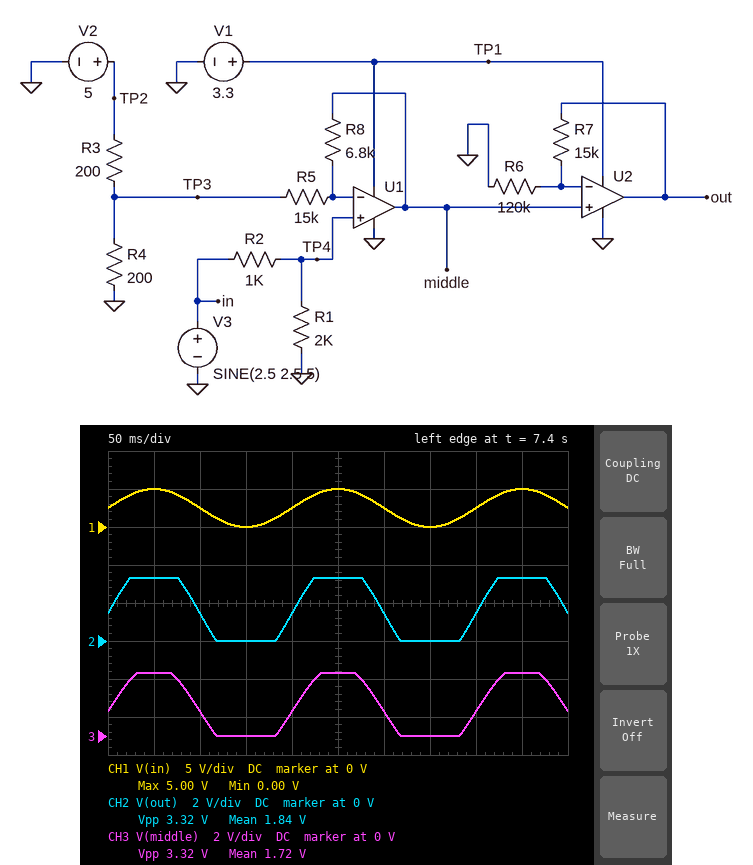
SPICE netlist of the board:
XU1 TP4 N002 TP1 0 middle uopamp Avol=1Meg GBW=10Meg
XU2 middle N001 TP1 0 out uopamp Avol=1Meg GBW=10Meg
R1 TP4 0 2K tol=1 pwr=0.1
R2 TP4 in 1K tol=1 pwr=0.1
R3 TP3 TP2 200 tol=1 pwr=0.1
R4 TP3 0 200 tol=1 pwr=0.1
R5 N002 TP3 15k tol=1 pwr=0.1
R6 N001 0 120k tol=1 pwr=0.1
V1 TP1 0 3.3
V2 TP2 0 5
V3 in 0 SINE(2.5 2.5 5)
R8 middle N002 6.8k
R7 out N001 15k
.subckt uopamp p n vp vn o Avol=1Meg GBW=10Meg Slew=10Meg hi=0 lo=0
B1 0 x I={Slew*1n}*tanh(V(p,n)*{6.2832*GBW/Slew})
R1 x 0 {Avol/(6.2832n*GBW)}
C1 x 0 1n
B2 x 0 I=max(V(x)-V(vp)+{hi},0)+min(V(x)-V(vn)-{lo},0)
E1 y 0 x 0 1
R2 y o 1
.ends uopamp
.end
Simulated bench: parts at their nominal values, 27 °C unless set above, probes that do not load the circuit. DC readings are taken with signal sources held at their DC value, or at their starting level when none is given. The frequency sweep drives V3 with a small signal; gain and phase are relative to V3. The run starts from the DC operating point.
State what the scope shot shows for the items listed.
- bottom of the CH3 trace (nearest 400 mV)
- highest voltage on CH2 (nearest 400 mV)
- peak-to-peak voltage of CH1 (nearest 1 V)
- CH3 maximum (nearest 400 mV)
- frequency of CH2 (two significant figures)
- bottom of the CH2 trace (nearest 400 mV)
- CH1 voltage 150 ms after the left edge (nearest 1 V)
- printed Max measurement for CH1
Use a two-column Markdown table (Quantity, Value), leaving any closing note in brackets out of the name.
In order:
| Quantity | Value |
|---|---|
| bottom of the CH3 trace | 0 V |
| highest voltage on CH2 | 3.2 V |
| peak-to-peak voltage of CH1 | 5 V |
| CH3 maximum | 3.2 V |
| frequency of CH2 | 5.0 Hz |
| bottom of the CH2 trace | 0 V |
| CH1 voltage 150 ms after the left edge | 0 V |
| printed Max measurement for CH1 | 5.00 V |
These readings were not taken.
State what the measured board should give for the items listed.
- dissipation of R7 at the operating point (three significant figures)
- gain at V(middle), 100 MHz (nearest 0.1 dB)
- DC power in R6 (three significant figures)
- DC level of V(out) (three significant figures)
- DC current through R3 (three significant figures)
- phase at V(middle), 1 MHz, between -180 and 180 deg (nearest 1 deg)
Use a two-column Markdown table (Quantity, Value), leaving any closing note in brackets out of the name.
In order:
| Quantity | Value |
|---|---|
| dissipation of R7 at the operating point | 1.74 µW |
| gain at V(middle), 100 MHz | -23.5 dB |
| DC power in R6 | 13.9 µW |
| DC level of V(out) | 1.45 V |
| DC current through R3 | 12.5 mA |
| phase at V(middle), 1 MHz, between -180 and 180 deg | -8 deg |
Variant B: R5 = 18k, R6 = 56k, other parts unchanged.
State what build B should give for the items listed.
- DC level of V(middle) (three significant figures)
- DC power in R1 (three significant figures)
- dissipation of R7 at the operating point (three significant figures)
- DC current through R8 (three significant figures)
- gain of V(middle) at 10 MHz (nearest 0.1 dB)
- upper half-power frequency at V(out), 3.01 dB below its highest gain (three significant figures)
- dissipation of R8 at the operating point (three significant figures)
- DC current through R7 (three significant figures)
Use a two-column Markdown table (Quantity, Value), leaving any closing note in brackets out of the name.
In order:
| Quantity | Value |
|---|---|
| DC level of V(middle) | 1.35 V |
| DC power in R1 | 1.39 mW |
| dissipation of R7 at the operating point | 8.76 µW |
| DC current through R8 | 46.0 µA |
| gain of V(middle) at 10 MHz | -5.4 dB |
| upper half-power frequency at V(out), 3.01 dB below its highest gain | 4.87 MHz |
| dissipation of R8 at the operating point | 14.4 µW |
| DC current through R7 | 24.2 µA |
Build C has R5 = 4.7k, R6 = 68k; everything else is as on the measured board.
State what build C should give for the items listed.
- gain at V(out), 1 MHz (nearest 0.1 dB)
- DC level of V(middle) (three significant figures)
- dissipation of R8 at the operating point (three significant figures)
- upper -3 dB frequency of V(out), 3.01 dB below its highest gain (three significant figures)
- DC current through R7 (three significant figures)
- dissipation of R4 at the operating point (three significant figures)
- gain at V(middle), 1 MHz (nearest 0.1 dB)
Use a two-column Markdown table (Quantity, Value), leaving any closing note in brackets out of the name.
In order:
| Quantity | Value |
|---|---|
| gain at V(out), 1 MHz | 5.6 dB |
| DC level of V(middle) | 486 mV |
| dissipation of R8 at the operating point | 205 µW |
| upper -3 dB frequency of V(out), 3.01 dB below its highest gain | 3.46 MHz |
| DC current through R7 | 7.15 µA |
| dissipation of R4 at the operating point | 30.8 mW |
| gain at V(middle), 1 MHz | 3.9 dB |
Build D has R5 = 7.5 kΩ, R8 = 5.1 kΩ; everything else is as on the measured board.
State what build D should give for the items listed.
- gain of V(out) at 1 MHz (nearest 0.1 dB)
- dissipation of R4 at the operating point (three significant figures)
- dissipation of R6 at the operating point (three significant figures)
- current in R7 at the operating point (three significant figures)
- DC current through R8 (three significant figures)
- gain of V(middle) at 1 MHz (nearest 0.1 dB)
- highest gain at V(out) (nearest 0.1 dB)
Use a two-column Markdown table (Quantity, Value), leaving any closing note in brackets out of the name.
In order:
| Quantity | Value |
|---|---|
| gain of V(out) at 1 MHz | 1.8 dB |
| dissipation of R4 at the operating point | 31.0 mW |
| dissipation of R6 at the operating point | 10.2 µW |
| current in R7 at the operating point | 9.23 µA |
| DC current through R8 | 110 µA |
| gain of V(middle) at 1 MHz | 0.8 dB |
| highest gain at V(out) | 2.0 dB |
